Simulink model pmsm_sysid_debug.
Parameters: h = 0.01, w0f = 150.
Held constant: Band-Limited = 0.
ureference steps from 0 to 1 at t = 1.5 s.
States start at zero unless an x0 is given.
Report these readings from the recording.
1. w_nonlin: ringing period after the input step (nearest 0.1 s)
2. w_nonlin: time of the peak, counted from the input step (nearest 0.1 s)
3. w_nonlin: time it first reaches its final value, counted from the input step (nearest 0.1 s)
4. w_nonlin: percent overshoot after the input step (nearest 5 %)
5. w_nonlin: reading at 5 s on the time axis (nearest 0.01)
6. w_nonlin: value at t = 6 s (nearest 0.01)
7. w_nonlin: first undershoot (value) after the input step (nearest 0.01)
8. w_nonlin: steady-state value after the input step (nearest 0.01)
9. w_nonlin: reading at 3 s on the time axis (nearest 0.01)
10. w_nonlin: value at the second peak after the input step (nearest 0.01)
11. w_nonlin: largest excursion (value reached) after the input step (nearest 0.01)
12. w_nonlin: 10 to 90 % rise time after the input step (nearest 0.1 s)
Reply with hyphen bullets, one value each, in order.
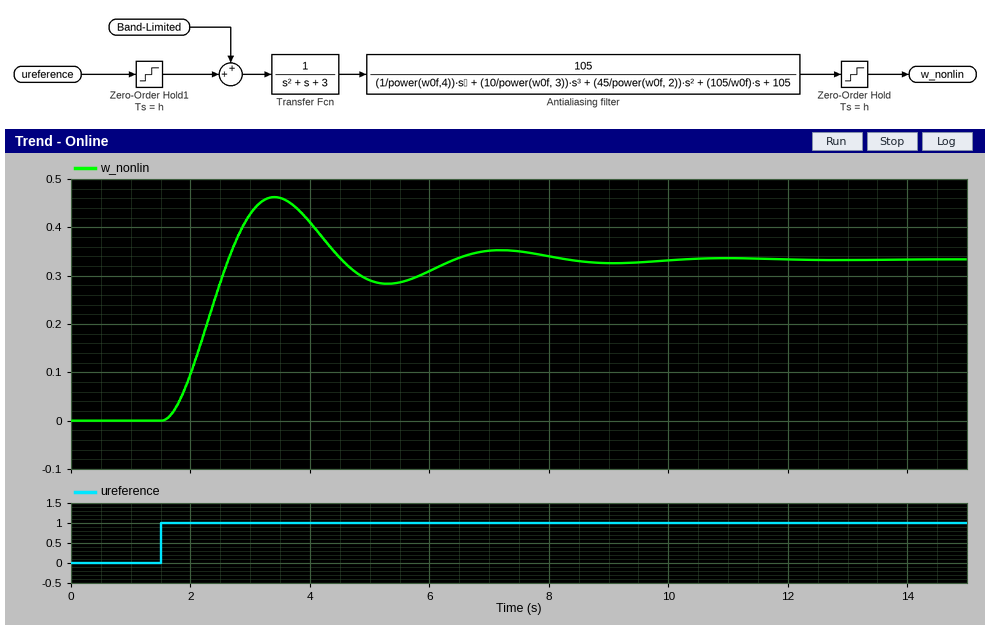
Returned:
- 3.8 s
- 1.9 s
- 1.1 s
- 40 %
- 0.29
- 0.31
- 0.28
- 0.33
- 0.43
- 0.35
- 0.46
- 0.8 s
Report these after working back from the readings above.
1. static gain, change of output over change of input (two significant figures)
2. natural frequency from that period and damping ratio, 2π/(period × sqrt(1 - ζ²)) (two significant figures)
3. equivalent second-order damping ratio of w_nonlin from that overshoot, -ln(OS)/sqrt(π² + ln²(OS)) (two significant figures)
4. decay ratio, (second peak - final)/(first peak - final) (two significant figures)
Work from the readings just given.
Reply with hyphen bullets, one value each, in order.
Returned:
- 0.33
- 1.7 rad/s
- 0.28
- 0.15
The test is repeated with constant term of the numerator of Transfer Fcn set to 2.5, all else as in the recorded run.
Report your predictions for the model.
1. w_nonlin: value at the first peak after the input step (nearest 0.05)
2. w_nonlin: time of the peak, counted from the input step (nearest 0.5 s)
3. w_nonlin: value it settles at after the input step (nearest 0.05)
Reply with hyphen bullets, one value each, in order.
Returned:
- 1.15
- 2.0 s
- 0.85
